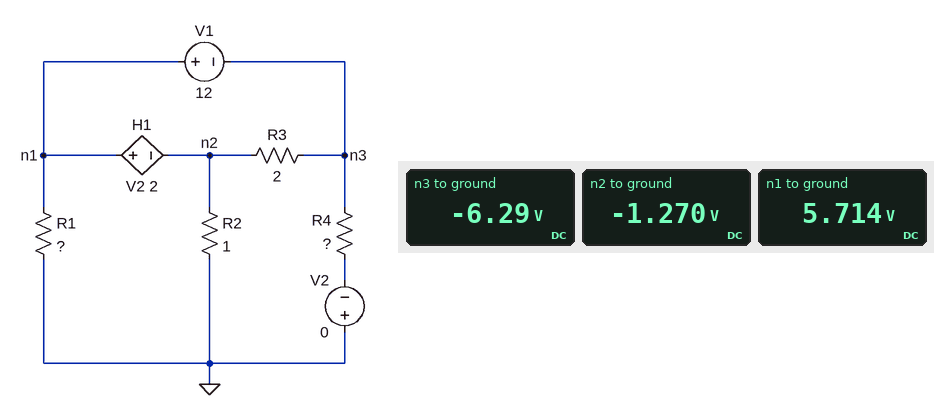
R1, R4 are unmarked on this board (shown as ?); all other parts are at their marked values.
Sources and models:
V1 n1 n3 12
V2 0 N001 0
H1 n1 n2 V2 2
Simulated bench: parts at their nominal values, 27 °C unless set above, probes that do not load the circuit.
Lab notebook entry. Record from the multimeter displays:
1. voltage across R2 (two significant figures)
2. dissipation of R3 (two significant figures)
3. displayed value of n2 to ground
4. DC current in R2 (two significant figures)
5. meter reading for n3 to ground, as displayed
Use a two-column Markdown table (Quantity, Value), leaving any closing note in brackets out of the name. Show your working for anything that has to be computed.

| Quantity | Value |
|---|---|
| voltage across R2 | 0 V - (-1.27 V) = 1.3 V |
| dissipation of R3 | (-1.27 V - (-6.29 V))^2 / 2 Ω = 13 W |
| displayed value of n2 to ground | -1.270 V |
| DC current in R2 | (0 V - (-1.27 V)) / 1 Ω = 1.3 A |
| meter reading for n3 to ground, as displayed | -6.29 V |
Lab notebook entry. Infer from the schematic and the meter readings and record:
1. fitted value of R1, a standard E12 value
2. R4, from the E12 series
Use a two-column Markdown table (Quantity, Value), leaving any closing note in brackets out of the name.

| Quantity | Value |
|---|---|
| fitted value of R1, a standard E12 value | 1.2 Ω |
| R4, from the E12 series | 1.8 Ω |
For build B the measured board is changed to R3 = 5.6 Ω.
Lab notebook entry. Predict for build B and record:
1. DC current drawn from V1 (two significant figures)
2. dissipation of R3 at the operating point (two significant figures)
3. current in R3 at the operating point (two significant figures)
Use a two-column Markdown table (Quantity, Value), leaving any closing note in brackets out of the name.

| Quantity | Value |
|---|---|
| DC current drawn from V1 | 4.4 A |
| dissipation of R3 at the operating point | 4.5 W |
| current in R3 at the operating point | 900 mA |
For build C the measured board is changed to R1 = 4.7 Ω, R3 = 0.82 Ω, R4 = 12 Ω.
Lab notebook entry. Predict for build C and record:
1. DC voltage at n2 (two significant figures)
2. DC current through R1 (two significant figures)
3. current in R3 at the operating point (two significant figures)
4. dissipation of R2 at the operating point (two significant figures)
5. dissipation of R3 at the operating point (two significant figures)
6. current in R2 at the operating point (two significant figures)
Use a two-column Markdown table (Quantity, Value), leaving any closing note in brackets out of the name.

| Quantity | Value |
|---|---|
| DC voltage at n2 | 390 mV |
| DC current through R1 | 440 mA |
| current in R3 at the operating point | 13 A |
| dissipation of R2 at the operating point | 150 mW |
| dissipation of R3 at the operating point | 130 W |
| current in R2 at the operating point | 390 mA |
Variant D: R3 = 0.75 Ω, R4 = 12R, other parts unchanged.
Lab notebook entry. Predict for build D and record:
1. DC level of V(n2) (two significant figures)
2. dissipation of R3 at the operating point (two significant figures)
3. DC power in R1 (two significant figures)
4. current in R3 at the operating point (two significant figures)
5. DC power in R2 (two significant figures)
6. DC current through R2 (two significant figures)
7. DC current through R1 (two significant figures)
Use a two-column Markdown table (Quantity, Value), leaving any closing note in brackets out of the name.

| Quantity | Value |
|---|---|
| DC level of V(n2) | -320 mV |
| dissipation of R3 at the operating point | 140 W |
| DC power in R1 | 1.7 W |
| current in R3 at the operating point | 14 A |
| DC power in R2 | 100 mW |
| DC current through R2 | 320 mA |
| DC current through R1 | 1.2 A |
